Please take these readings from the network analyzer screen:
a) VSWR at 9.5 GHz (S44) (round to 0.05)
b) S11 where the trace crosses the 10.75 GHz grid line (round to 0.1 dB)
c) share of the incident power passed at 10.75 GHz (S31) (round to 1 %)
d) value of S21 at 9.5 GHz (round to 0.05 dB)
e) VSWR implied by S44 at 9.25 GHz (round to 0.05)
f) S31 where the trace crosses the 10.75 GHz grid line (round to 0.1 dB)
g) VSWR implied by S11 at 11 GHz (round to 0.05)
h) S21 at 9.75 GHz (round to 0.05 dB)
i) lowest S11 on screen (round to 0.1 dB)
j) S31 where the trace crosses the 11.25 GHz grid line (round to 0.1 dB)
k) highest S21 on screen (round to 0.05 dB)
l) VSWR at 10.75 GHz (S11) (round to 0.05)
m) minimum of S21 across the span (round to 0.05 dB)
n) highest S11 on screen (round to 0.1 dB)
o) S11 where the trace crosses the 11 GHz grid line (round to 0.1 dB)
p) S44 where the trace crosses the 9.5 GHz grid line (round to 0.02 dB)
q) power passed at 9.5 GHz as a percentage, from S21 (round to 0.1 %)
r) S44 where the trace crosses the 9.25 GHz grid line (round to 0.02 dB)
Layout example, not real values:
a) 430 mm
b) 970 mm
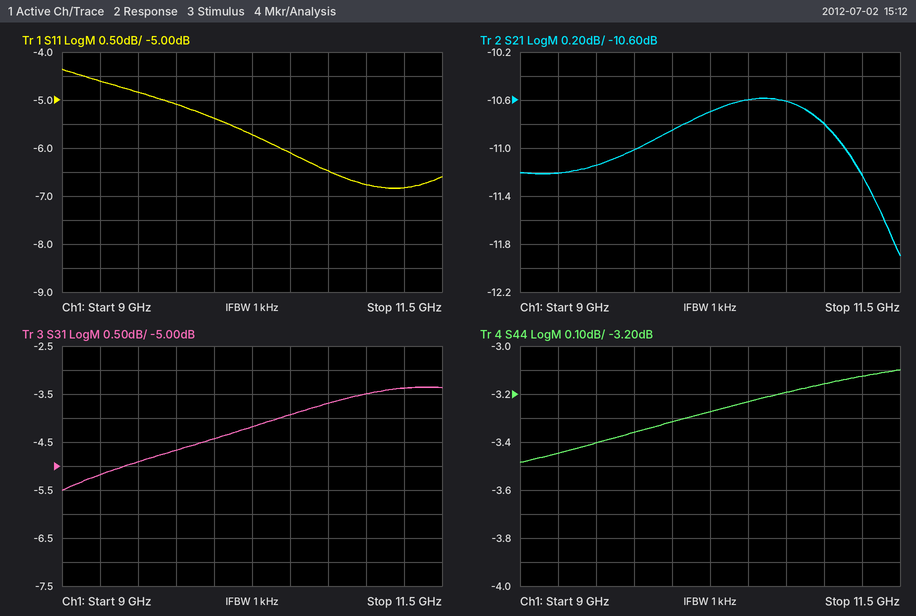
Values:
a) 5.15
b) -6.5 dB
c) 43 %
d) -11.15 dB
e) 5.10
f) -3.7 dB
g) 2.70
h) -11.00 dB
i) -6.8 dB
j) -3.4 dB
k) -10.60 dB
l) 2.80
m) -11.90 dB
n) -4.4 dB
o) -6.8 dB
p) -3.40 dB
q) 7.7 %
r) -3.44 dB
